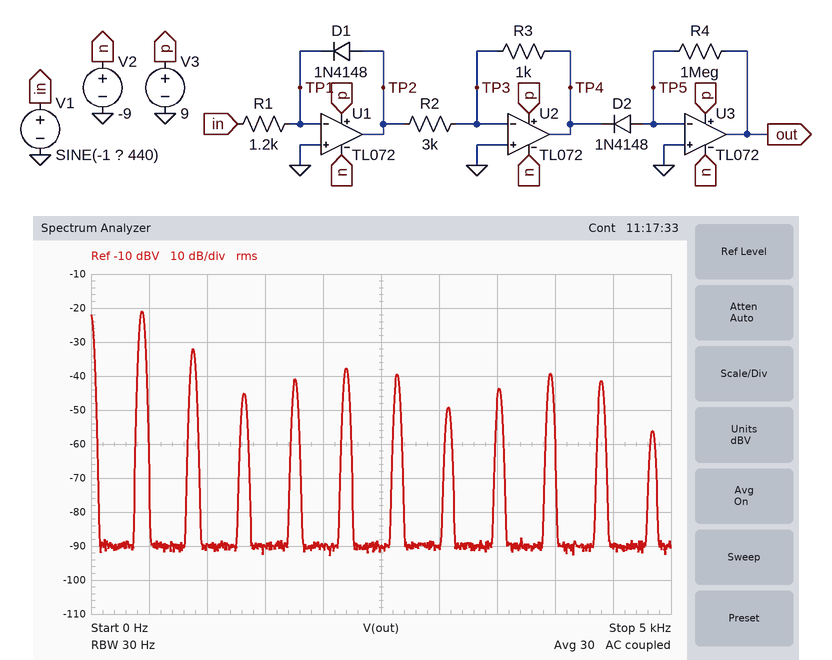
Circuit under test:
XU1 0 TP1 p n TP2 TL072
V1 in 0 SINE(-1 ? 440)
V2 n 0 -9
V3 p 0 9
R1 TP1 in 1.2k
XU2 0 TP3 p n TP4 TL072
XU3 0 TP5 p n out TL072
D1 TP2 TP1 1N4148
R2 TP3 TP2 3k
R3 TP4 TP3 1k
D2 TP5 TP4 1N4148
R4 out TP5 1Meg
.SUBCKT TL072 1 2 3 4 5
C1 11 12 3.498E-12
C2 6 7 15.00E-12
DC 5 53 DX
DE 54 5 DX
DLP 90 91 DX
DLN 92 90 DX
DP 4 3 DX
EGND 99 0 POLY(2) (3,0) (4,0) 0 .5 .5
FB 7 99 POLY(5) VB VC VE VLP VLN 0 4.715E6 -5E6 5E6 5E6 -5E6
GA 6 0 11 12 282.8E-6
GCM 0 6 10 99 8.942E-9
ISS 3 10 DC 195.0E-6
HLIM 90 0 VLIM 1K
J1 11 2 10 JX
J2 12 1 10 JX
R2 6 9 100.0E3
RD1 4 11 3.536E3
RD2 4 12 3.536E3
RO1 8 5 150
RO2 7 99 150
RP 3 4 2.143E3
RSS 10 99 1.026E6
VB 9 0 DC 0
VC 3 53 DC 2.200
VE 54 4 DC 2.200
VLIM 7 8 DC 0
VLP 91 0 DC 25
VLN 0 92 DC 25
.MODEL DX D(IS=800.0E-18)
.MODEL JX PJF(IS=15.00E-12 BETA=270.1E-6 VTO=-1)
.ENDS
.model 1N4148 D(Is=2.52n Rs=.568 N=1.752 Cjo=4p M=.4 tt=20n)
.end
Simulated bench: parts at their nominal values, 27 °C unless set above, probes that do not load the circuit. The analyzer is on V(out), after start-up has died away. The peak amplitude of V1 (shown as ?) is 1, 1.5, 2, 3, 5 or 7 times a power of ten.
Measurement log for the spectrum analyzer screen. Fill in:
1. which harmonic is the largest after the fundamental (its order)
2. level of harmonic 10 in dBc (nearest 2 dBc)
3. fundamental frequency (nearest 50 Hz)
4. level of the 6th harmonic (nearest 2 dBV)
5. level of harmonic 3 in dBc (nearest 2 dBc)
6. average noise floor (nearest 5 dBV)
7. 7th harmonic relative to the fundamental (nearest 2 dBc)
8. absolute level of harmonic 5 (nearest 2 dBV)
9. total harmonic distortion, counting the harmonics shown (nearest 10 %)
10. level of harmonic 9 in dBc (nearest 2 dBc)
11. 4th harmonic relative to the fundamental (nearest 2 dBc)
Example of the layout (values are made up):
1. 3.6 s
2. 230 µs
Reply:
1. 2
2. -20 dBc
3. 450 Hz
4. -40 dBV
5. -24 dBc
6. -90 dBV
7. -28 dBc
8. -38 dBV
9. 40 %
10. -18 dBc
11. -20 dBc
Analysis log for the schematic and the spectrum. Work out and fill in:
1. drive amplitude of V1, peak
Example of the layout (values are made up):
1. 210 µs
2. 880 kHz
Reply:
1. 1.5 V
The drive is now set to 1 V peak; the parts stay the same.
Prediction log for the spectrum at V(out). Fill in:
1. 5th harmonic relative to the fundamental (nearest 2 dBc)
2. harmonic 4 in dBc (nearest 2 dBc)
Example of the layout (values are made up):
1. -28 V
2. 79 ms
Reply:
1. -24 dBc
2. -22 dBc
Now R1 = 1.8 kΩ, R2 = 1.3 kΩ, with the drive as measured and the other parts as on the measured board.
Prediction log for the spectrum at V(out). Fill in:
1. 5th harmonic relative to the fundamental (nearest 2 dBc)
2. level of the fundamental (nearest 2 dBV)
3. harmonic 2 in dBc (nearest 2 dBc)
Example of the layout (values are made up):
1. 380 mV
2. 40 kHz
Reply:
1. -12 dBc
2. 8 dBV
3. -4 dBc
